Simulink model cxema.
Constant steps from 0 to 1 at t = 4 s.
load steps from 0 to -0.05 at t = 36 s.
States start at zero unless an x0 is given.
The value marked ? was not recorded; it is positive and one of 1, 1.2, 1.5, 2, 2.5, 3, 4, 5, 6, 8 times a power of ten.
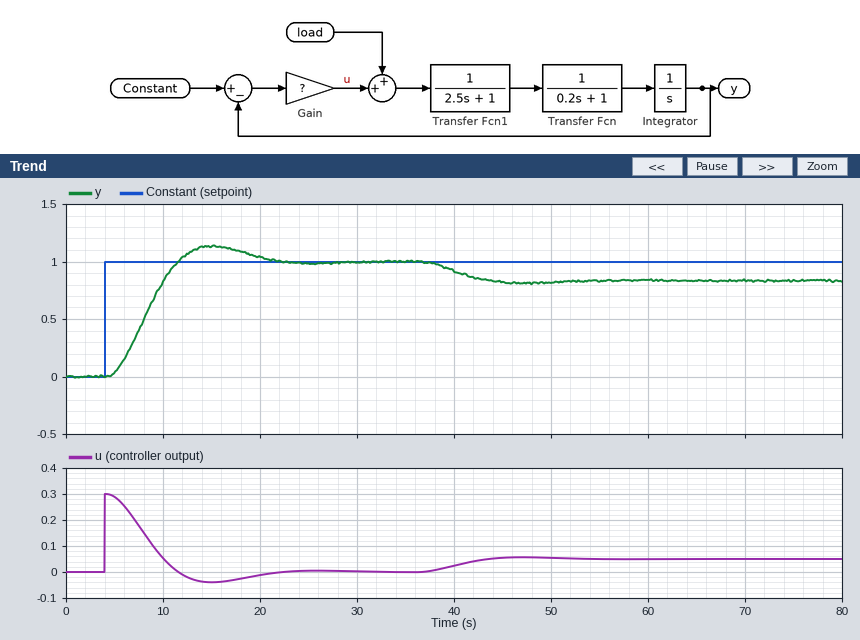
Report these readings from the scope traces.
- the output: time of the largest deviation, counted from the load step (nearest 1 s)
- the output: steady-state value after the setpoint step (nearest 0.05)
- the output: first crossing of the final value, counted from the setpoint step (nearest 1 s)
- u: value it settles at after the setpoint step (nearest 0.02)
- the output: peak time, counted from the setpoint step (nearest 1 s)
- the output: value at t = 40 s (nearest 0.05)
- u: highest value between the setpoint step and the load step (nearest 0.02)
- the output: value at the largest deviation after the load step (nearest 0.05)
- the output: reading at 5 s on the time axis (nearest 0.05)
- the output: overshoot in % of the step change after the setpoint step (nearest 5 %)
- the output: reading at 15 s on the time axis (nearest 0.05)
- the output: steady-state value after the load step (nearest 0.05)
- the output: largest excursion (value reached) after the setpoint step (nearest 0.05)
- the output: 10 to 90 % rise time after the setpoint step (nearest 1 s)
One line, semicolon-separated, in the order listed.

11 s; 1.00; 8 s; 0.00; 11 s; 0.90; 0.30; 0.80; 0.05; 15 %; 1.15; 0.85; 1.15; 5 s
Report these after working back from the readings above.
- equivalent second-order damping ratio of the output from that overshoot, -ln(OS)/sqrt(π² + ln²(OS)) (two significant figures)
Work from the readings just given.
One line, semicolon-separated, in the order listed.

0.52
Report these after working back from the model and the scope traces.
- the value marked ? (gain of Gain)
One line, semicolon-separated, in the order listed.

0.3
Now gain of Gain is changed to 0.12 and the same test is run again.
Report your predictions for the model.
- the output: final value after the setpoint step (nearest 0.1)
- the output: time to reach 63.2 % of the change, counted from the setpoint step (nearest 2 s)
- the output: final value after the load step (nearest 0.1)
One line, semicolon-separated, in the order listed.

1.0; 10 s; 0.6
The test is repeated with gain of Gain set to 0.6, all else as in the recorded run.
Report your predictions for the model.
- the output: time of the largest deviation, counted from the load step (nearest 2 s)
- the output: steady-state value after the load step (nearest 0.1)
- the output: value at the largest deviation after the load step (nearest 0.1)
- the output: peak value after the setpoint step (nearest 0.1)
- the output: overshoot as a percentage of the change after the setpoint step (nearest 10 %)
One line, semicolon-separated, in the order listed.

8 s; 0.9; 0.9; 1.3; 30 %
